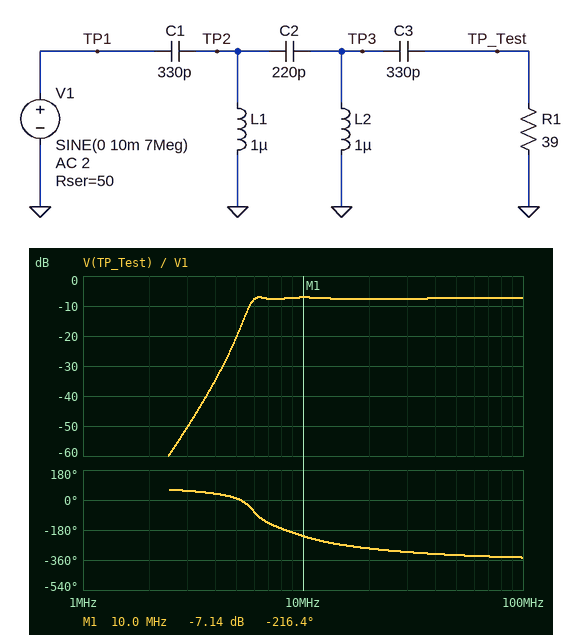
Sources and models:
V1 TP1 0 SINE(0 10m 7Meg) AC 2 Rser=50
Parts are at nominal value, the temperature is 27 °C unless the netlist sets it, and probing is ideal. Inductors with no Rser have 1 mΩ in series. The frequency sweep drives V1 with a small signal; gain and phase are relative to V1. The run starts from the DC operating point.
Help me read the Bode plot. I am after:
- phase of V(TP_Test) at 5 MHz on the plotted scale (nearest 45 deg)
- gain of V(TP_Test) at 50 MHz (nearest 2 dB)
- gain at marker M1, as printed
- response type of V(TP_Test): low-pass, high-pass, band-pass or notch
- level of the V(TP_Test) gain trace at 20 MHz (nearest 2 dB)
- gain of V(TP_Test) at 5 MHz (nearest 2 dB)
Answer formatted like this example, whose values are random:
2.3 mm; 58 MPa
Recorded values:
0 deg; -8 dB; -7.14 dB; high-pass; -8 dB; -20 dB
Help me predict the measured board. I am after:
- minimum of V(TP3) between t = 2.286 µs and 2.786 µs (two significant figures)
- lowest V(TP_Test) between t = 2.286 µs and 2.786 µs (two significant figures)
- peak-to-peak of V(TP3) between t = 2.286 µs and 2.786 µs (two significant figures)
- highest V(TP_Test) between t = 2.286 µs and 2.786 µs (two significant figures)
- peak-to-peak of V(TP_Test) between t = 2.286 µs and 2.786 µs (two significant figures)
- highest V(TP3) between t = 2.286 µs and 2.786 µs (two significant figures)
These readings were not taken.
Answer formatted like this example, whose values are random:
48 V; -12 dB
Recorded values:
-8.5 mV; -4.2 mV; 17 mV; 4.2 mV; 8.3 mV; 8.5 mV
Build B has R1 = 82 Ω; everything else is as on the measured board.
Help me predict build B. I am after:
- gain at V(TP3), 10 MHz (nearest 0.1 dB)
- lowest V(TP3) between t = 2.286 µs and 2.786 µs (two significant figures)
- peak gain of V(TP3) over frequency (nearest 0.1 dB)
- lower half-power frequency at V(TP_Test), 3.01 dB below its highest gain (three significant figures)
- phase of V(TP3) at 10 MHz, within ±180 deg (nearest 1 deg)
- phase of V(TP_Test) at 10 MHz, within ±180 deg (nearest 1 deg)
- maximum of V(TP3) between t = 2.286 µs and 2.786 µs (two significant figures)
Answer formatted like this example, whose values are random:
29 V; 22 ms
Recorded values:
-3.0 dB; -8.2 mV; -1.5 dB; 5.90 MHz; 112 deg; 142 deg; 8.2 mV
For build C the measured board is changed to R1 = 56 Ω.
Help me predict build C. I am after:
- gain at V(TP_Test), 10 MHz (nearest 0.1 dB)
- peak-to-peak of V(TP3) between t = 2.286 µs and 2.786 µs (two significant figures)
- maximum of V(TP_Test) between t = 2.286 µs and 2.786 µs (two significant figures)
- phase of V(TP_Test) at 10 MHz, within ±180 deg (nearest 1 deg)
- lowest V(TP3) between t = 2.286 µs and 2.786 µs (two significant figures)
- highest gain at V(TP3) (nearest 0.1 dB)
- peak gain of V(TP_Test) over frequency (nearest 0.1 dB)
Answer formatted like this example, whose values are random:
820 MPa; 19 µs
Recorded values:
-5.6 dB; 16 mV; 5.2 mV; 143 deg; -8.2 mV; -1.1 dB; -5.5 dB
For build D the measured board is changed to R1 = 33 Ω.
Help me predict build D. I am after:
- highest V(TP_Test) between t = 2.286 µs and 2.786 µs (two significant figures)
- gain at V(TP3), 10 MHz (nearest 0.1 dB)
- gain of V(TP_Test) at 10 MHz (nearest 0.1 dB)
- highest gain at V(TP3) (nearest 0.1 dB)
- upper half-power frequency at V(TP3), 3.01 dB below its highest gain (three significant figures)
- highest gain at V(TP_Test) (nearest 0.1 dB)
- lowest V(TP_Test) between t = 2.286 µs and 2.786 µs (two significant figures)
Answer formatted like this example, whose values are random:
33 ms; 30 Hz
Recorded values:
3.7 mV; -3.0 dB; -8.0 dB; 0.4 dB; 9.39 MHz; -7.8 dB; -3.7 mV
